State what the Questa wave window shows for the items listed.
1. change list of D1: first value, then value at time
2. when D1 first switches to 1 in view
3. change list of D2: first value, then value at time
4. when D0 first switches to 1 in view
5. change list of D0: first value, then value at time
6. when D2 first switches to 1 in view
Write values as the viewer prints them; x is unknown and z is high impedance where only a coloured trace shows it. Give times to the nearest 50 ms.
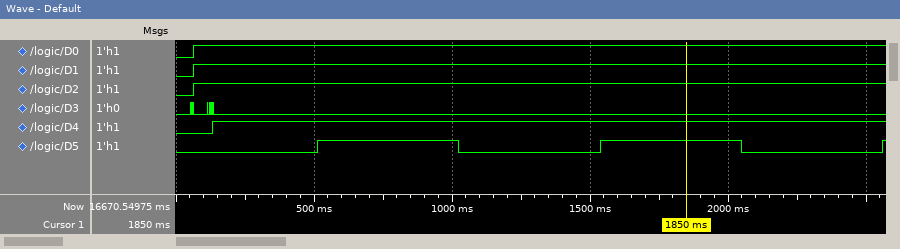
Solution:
0, 1 at 50 ms
50 ms
0, 1 at 50 ms
50 ms
0, 1 at 50 ms
50 ms
